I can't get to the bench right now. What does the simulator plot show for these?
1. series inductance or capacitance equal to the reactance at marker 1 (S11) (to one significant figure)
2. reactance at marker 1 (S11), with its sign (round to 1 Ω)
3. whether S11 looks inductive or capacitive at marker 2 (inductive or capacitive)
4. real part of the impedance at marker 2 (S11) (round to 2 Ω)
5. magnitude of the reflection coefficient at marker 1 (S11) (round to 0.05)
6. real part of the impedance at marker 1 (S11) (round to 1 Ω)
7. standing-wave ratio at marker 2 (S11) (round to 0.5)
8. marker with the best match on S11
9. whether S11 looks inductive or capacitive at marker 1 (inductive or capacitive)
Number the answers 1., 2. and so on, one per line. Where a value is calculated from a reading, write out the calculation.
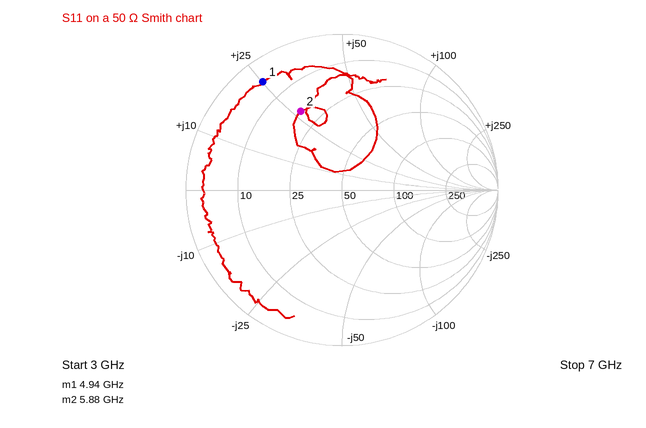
1. L = 25 Ω/(2π × 4.94 GHz) ≈ 805 pH, so 800 pH to one significant figure
2. +25 Ω
3. inductive
4. 18 Ω
5. 0.85
6. 5 Ω
7. 3.5
8. marker 2
9. inductive
